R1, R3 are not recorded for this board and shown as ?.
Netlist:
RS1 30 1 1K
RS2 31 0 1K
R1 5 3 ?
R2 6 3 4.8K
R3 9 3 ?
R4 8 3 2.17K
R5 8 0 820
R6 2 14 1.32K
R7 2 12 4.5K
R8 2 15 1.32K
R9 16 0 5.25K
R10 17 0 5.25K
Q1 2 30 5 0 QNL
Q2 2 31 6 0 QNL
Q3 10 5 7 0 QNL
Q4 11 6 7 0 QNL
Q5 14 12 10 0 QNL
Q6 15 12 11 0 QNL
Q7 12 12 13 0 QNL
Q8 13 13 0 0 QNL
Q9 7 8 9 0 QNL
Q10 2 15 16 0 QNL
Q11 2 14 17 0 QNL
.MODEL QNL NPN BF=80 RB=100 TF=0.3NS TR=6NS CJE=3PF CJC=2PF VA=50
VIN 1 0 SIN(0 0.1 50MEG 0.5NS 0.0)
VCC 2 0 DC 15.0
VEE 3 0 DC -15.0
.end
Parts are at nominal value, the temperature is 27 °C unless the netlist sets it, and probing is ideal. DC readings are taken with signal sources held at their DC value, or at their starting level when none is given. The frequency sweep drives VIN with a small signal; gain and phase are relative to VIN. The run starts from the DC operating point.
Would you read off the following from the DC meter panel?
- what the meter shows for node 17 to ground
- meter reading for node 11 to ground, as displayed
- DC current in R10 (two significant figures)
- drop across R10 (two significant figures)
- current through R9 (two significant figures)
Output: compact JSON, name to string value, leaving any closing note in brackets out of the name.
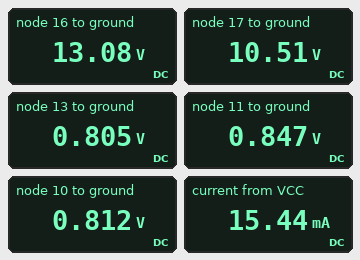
{"what the meter shows for node 17 to ground": "10.51 V", "meter reading for node 11 to ground, as displayed": "0.847 V", "DC current in R10": "2.0 mA", "drop across R10": "11 V", "current through R9": "2.5 mA"}
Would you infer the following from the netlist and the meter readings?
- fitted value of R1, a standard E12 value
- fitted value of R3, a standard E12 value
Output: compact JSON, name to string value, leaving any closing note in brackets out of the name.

{"fitted value of R1, a standard E12 value": "10 kΩ", "fitted value of R3, a standard E12 value": "2.7 kΩ"}
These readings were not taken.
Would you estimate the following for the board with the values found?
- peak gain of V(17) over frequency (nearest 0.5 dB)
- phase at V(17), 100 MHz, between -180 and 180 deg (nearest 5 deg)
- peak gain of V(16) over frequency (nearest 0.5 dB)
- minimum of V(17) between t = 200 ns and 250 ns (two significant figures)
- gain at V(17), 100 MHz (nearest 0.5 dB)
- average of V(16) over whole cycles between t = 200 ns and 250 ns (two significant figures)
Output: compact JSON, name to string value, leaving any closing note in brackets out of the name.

{"peak gain of V(17) over frequency": "29.5 dB", "phase at V(17), 100 MHz, between -180 and 180 deg": "-30 deg", "peak gain of V(16) over frequency": "29.5 dB", "minimum of V(17) between t = 200 ns and 250 ns": "9.8 V", "gain at V(17), 100 MHz": "11.0 dB", "average of V(16) over whole cycles between t = 200 ns and 250 ns": "12 V"}
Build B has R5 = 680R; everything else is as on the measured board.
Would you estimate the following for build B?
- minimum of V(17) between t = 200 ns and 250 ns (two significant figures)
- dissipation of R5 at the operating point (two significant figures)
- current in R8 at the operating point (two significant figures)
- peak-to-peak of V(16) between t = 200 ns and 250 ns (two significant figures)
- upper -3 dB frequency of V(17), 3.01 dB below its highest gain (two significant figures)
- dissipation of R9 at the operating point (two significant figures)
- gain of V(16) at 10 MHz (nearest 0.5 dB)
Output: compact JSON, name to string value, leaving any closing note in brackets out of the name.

{"minimum of V(17) between t = 200 ns and 250 ns": "9.5 V", "dissipation of R5 at the operating point": "19 mW", "current in R8 at the operating point": "890 µA", "peak-to-peak of V(16) between t = 200 ns and 250 ns": "3.1 V", "upper -3 dB frequency of V(17), 3.01 dB below its highest gain": "45 MHz", "dissipation of R9 at the operating point": "32 mW", "gain of V(16) at 10 MHz": "30.0 dB"}
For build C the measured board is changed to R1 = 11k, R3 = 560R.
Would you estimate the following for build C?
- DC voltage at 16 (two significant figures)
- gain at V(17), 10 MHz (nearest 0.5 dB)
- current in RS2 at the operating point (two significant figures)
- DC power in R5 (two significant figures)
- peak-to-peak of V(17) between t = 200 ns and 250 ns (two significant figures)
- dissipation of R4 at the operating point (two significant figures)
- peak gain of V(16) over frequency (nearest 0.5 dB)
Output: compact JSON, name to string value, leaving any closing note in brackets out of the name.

{"DC voltage at 16": "8.1 V", "gain at V(17), 10 MHz": "19.0 dB", "current in RS2 at the operating point": "29 µA", "DC power in R5": "22 mW", "peak-to-peak of V(17) between t = 200 ns and 250 ns": "520 mV", "dissipation of R4 at the operating point": "53 mW", "peak gain of V(16) over frequency": "41.5 dB"}
